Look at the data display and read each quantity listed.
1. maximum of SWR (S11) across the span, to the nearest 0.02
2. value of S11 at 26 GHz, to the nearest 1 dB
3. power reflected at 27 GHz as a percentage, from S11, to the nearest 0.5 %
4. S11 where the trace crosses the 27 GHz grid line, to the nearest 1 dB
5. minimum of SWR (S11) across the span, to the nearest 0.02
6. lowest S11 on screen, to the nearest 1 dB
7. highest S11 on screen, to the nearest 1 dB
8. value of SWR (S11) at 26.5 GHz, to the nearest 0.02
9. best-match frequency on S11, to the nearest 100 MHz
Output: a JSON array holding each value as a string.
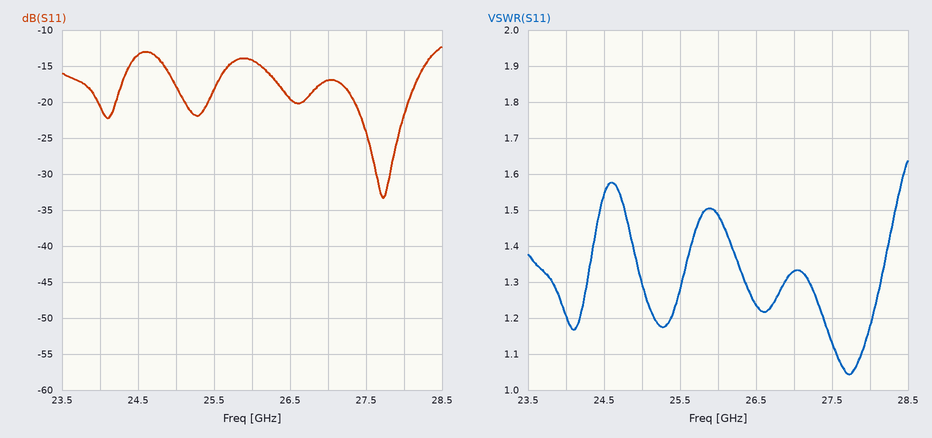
["1.64", "-14 dB", "2.0 %", "-17 dB", "1.04", "-33 dB", "-12 dB", "1.24", "27.7 GHz"]
